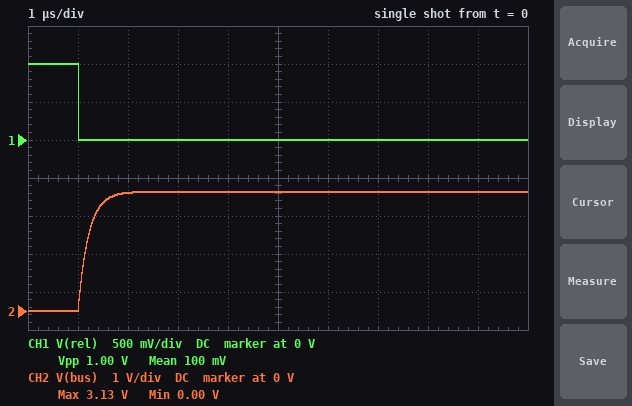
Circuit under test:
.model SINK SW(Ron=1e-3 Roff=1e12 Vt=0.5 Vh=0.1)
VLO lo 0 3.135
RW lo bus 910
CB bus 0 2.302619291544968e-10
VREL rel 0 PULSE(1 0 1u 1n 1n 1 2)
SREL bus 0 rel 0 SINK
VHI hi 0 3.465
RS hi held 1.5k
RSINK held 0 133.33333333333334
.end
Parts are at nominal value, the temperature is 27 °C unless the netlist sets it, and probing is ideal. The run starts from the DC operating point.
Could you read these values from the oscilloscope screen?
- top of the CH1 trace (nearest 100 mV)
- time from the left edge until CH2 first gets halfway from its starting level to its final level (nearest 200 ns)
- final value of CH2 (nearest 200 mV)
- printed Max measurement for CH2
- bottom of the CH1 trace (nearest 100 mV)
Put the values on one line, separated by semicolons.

1.0 V; 1.2 µs; 3.2 V; 3.13 V; 0 V
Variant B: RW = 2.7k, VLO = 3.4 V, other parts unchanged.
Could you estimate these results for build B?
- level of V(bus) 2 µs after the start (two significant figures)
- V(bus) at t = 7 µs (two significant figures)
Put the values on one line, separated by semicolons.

2.7 V; 3.4 V
